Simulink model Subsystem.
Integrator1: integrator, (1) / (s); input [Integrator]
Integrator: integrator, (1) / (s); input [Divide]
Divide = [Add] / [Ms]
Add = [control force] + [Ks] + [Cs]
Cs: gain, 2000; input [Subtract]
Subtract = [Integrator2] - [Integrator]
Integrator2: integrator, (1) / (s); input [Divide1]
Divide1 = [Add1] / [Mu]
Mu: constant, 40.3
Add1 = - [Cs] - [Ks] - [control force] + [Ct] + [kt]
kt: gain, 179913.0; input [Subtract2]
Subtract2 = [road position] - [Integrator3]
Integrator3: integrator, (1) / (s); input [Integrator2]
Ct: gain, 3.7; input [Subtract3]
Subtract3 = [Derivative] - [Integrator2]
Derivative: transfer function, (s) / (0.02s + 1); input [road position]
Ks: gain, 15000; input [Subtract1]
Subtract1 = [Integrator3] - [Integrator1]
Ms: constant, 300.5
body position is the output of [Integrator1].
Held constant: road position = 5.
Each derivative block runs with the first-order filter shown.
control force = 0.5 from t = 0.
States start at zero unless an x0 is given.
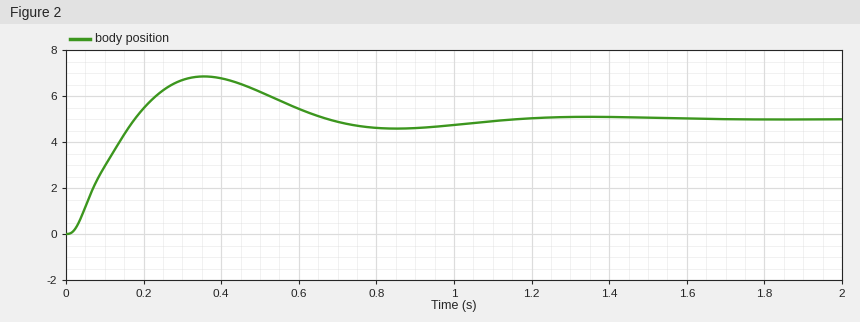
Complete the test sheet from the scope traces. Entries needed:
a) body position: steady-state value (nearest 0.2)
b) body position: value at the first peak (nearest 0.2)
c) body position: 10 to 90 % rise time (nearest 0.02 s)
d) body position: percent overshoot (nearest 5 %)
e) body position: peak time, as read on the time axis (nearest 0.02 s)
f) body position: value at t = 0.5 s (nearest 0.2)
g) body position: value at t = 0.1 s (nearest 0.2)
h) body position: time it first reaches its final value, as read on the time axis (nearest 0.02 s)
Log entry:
5.0
6.8
0.12 s
35 %
0.36 s
6.2
3.0
0.18 s
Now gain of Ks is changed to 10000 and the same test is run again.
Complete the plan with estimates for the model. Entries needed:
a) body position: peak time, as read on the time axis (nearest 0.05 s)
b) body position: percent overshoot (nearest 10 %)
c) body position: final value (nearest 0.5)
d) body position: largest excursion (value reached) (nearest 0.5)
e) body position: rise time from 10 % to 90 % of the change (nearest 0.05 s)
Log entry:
0.40 s
30 %
5.0
6.5
0.15 s
